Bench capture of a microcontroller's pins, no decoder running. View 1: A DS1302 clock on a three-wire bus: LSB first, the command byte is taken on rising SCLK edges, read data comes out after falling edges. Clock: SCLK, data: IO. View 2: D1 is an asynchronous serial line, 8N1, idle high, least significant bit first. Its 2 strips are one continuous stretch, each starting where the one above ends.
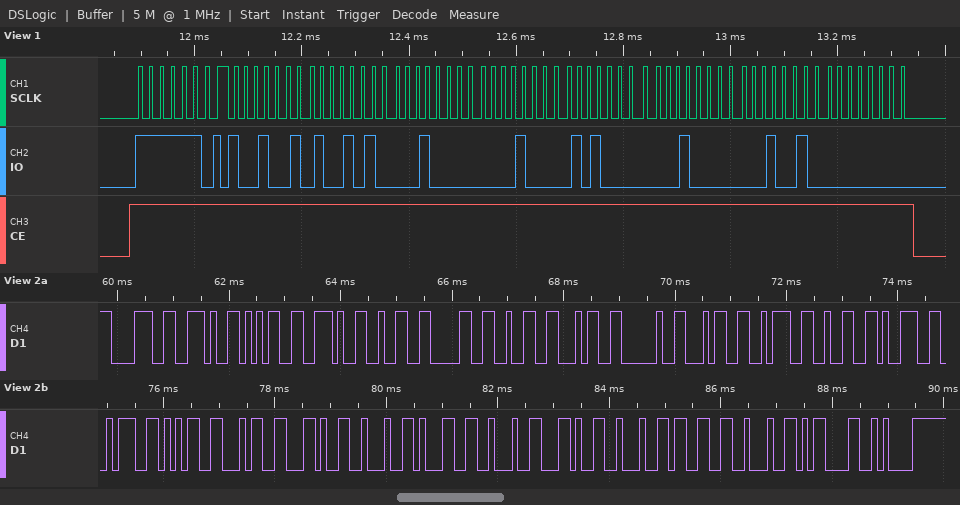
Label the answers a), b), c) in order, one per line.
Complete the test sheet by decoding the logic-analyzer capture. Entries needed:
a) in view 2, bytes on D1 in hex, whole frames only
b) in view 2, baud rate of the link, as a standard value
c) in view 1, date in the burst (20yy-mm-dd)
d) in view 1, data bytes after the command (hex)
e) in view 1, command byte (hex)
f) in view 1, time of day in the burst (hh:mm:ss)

a) 38 2E 35 2E 32 30 32 34 20 34 3A 32 39 3A 35 34 2C 22 31 22 2C 22 33 22 0D 0A
b) 9600 baud
c) 2024-05-08
d) 49 29 04 08 05 04 24 00
e) 0xBF
f) 04:29:49
